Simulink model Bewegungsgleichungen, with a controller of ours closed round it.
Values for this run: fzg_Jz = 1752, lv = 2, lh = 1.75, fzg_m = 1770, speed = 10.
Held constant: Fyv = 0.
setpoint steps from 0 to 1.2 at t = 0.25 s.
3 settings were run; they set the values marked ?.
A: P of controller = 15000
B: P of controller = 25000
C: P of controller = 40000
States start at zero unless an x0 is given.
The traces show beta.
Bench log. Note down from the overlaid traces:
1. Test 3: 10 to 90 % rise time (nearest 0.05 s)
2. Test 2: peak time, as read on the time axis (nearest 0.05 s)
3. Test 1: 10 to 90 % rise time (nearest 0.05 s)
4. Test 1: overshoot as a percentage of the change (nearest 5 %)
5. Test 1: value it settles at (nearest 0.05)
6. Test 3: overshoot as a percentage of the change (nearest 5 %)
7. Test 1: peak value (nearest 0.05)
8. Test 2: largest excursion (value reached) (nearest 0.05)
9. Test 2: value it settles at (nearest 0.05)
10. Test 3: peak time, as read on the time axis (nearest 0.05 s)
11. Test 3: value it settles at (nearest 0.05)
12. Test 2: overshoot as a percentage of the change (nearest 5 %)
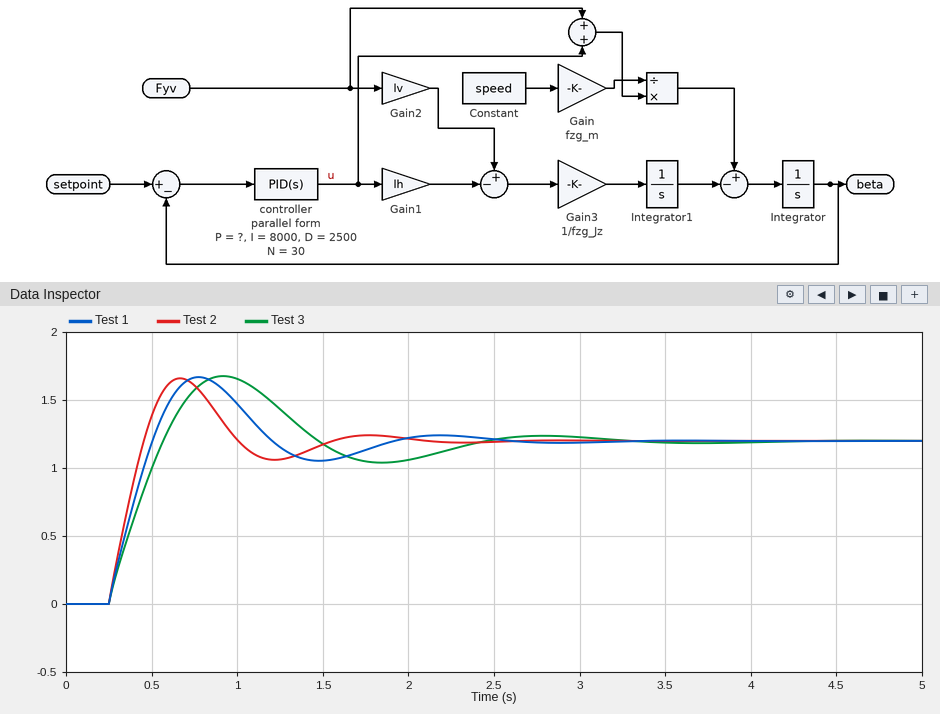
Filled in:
0.25 s
0.65 s
0.20 s
40 %
1.20
40 %
1.65
1.65
1.20
0.90 s
1.20
40 %
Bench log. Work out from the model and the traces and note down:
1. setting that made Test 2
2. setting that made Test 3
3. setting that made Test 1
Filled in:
C
A
B
